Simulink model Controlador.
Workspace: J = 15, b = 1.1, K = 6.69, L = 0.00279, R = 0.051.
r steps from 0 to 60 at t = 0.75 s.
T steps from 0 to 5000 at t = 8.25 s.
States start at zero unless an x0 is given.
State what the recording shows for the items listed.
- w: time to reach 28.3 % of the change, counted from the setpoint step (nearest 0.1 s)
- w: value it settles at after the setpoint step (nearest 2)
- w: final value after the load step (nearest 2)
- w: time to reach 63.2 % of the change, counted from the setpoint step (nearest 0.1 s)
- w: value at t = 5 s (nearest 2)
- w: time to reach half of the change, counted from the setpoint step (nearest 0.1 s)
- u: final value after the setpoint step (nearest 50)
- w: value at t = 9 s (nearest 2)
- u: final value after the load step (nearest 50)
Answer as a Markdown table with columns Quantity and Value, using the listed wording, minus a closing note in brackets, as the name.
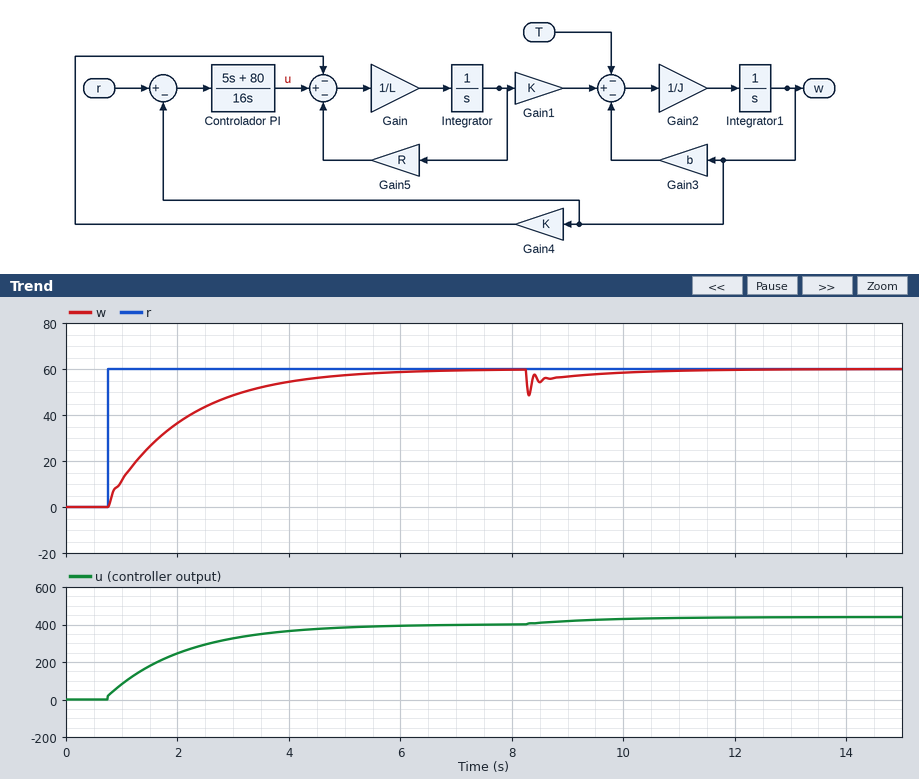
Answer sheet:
| Quantity | Value |
|---|---|
| w: time to reach 28.3 % of the change, counted from the setpoint step | 0.4 s |
| w: value it settles at after the setpoint step | 60 |
| w: final value after the load step | 60 |
| w: time to reach 63.2 % of the change, counted from the setpoint step | 1.3 s |
| w: value at t = 5 s | 58 |
| w: time to reach half of the change, counted from the setpoint step | 0.9 s |
| u: final value after the setpoint step | 400 |
| w: value at t = 9 s | 56 |
| u: final value after the load step | 450 |
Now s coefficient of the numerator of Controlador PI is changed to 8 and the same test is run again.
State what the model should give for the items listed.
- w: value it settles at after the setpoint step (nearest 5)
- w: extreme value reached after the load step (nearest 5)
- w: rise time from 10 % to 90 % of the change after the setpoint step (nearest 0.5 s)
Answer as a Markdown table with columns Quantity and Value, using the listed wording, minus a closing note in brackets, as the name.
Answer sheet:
| Quantity | Value |
|---|---|
| w: value it settles at after the setpoint step | 60 |
| w: extreme value reached after the load step | 50 |
| w: rise time from 10 % to 90 % of the change after the setpoint step | 3.0 s |
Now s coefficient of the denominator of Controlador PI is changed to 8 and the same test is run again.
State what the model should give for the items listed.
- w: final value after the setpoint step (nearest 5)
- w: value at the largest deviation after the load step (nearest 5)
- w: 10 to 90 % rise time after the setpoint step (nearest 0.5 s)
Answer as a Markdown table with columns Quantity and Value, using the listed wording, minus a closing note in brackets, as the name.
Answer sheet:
| Quantity | Value |
|---|---|
| w: final value after the setpoint step | 60 |
| w: value at the largest deviation after the load step | 50 |
| w: 10 to 90 % rise time after the setpoint step | 1.5 s |
